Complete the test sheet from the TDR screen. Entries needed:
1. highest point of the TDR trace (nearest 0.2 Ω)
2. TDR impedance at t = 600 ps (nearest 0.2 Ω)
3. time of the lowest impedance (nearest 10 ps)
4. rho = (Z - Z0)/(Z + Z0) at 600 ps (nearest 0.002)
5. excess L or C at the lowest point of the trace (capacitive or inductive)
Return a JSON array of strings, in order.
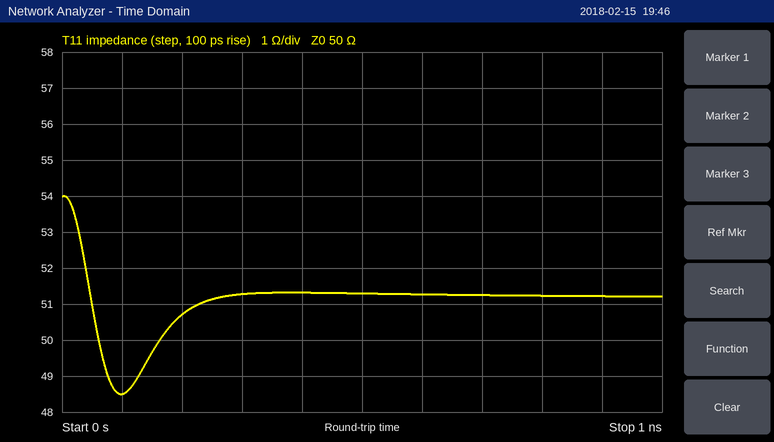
["54.0 Ω", "51.2 Ω", "100 ps", "+0.012", "capacitive"]
